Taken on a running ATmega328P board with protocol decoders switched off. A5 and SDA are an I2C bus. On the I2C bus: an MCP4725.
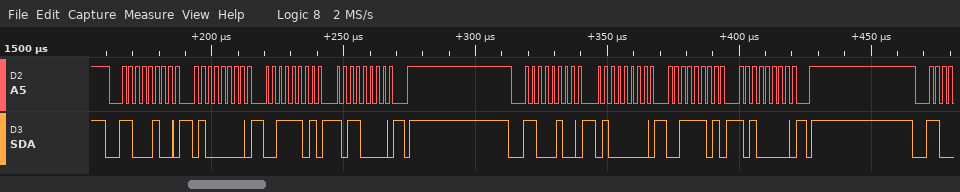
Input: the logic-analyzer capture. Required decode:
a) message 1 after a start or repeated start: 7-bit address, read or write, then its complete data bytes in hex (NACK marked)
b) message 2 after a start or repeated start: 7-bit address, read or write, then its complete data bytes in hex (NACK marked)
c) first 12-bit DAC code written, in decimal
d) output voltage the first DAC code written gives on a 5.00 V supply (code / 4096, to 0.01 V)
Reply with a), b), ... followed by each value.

a) 0x62 write: 40 3D B0
b) 0x62 write: 40 3D A0
c) 987
d) 1.20 V
